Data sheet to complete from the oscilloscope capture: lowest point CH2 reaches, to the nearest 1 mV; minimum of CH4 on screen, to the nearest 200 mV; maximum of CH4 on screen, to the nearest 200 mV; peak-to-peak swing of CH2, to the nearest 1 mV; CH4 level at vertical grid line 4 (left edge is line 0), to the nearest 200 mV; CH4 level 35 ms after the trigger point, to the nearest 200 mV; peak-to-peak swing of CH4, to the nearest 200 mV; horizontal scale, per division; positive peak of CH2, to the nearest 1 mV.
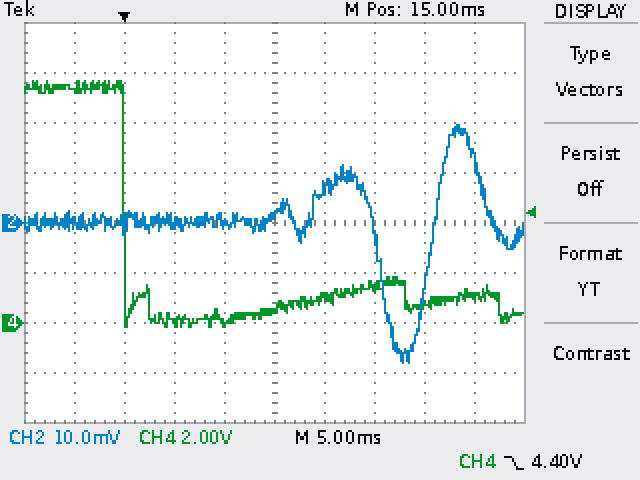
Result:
-28 mV
-200 mV
9.6 V
48 mV
0.0 V
1.0 V
9.8 V
5 ms
20 mV
